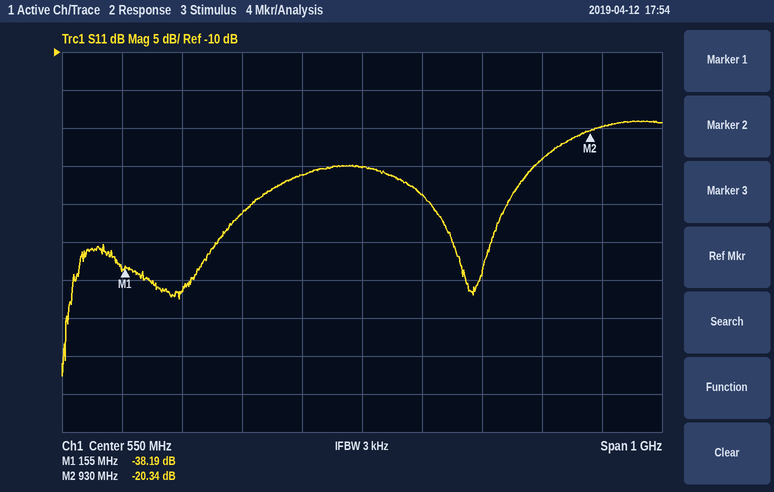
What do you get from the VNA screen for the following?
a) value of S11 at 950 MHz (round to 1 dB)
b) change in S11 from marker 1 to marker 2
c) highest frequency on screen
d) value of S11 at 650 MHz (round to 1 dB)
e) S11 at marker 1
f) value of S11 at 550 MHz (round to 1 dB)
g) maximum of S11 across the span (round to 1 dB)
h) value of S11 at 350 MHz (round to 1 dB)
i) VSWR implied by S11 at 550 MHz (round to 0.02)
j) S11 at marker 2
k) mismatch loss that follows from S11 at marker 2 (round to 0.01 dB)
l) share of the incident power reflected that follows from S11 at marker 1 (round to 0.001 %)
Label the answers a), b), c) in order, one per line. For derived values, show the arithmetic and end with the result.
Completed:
a) -20 dB
b) -20.34 − (-38.19) = 17.85 dB
c) 1.05 GHz
d) -29 dB
e) -38.19 dB
f) -25 dB
g) -19 dB
h) -31 dB
i) |Γ| = 10^(-25/20) = 0.0562; VSWR = (1 + 0.0562)/(1 − 0.0562) ≈ 1.12
j) -20.34 dB
k) −10 log10(1 − 10^(-20.34/10)) ≈ 0.04 dB
l) 10^(-38.19/10) ≈ 0.015 %
